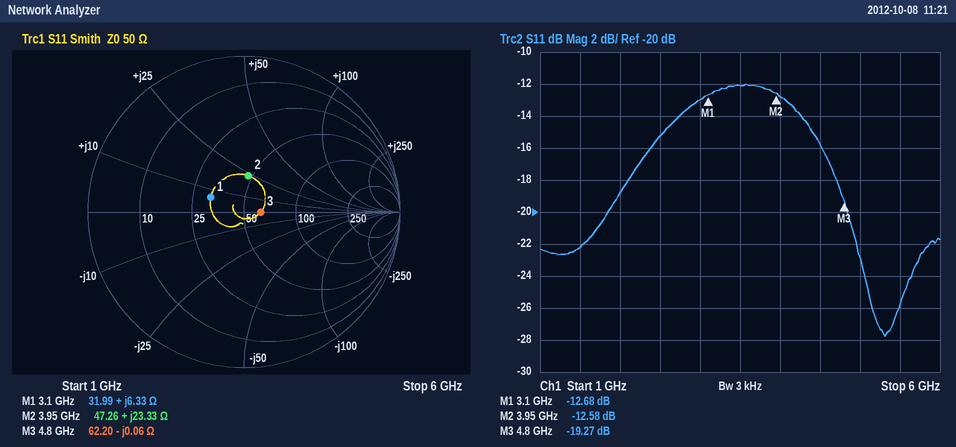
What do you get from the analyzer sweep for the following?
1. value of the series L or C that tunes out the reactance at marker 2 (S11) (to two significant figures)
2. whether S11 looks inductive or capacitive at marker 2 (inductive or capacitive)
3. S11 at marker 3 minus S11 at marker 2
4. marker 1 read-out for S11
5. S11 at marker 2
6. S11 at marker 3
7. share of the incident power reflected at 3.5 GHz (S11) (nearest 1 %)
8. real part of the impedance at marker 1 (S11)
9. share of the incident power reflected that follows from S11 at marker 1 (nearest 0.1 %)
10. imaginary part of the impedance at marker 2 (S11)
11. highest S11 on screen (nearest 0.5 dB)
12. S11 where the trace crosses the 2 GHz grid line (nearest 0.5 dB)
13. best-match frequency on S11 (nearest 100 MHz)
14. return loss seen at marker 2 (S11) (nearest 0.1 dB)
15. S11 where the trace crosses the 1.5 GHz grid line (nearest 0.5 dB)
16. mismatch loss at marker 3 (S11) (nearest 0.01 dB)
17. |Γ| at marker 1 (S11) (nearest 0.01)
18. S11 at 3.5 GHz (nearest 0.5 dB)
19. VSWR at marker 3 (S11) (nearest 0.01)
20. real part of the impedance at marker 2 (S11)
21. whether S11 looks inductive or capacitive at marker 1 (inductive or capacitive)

1.7 pF
inductive
-6.69 dB
-12.68 dB
-12.58 dB
-19.27 dB
6 %
31.99 Ω
5.4 %
+23.33 Ω
-12.0 dB
-19.0 dB
5.3 GHz
12.6 dB
-22.0 dB
0.05 dB
0.23
-12.0 dB
1.24
47.26 Ω
inductive
